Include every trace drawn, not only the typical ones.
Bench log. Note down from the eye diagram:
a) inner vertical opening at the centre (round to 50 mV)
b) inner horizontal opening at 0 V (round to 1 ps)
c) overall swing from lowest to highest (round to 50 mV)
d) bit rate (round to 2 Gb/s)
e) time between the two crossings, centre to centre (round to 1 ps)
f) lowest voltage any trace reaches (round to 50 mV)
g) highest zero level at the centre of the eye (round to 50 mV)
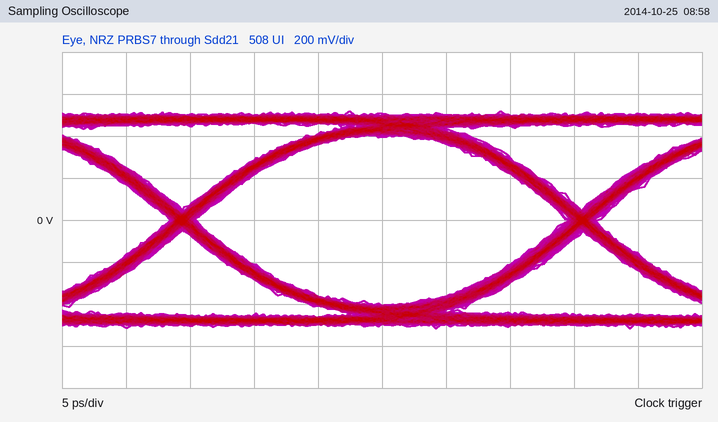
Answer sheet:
800 mV
29 ps
1.05 V
32 Gb/s
31 ps
-500 mV
-400 mV
